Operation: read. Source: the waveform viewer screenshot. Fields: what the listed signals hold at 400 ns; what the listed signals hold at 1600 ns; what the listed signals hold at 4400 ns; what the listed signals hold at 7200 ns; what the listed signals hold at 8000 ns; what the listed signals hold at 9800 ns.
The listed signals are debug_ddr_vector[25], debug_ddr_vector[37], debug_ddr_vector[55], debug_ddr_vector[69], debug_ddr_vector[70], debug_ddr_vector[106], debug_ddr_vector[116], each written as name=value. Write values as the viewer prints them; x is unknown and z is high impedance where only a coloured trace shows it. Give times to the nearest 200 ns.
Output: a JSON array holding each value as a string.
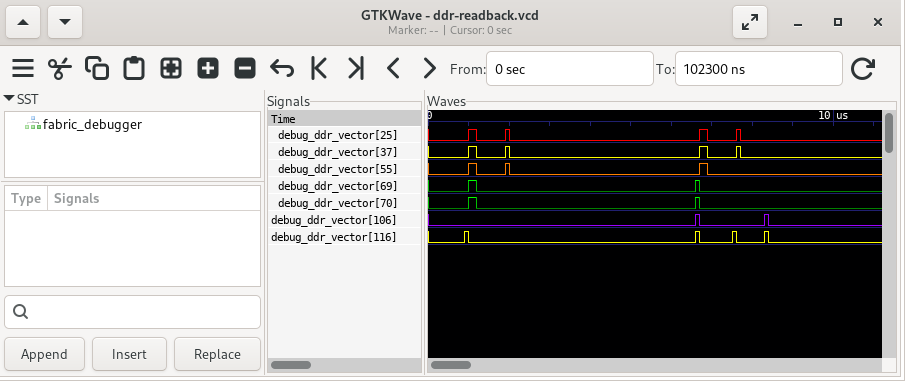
["debug_ddr_vector[25]=0, debug_ddr_vector[37]=0, debug_ddr_vector[55]=0, debug_ddr_vector[69]=0, debug_ddr_vector[70]=0, debug_ddr_vector[106]=0, debug_ddr_vector[116]=0", "debug_ddr_vector[25]=0, debug_ddr_vector[37]=0, debug_ddr_vector[55]=0, debug_ddr_vector[69]=0, debug_ddr_vector[70]=0, debug_ddr_vector[106]=0, debug_ddr_vector[116]=0", "debug_ddr_vector[25]=0, debug_ddr_vector[37]=0, debug_ddr_vector[55]=0, debug_ddr_vector[69]=0, debug_ddr_vector[70]=0, debug_ddr_vector[106]=0, debug_ddr_vector[116]=0", "debug_ddr_vector[25]=0, debug_ddr_vector[37]=0, debug_ddr_vector[55]=0, debug_ddr_vector[69]=0, debug_ddr_vector[70]=0, debug_ddr_vector[106]=0, debug_ddr_vector[116]=0", "debug_ddr_vector[25]=0, debug_ddr_vector[37]=0, debug_ddr_vector[55]=0, debug_ddr_vector[69]=0, debug_ddr_vector[70]=0, debug_ddr_vector[106]=0, debug_ddr_vector[116]=0", "debug_ddr_vector[25]=0, debug_ddr_vector[37]=0, debug_ddr_vector[55]=0, debug_ddr_vector[69]=0, debug_ddr_vector[70]=0, debug_ddr_vector[106]=0, debug_ddr_vector[116]=0"]
